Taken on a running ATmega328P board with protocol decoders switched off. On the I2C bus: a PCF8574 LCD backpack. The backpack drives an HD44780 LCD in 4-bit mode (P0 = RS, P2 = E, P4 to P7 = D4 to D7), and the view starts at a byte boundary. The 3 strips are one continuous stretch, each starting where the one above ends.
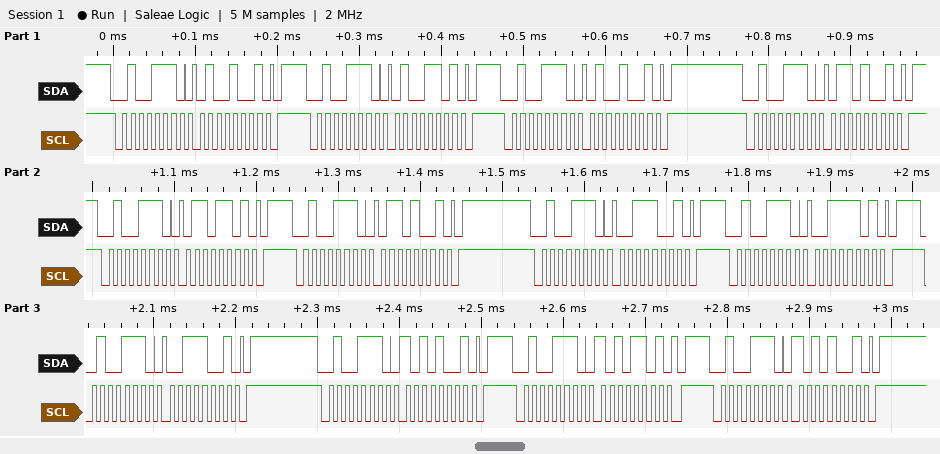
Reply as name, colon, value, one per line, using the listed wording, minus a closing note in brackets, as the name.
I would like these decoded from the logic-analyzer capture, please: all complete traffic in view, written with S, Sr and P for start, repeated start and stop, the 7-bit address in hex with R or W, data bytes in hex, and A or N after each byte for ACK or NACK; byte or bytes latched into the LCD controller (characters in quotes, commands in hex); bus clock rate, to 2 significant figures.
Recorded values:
all complete traffic in view, written with S, Sr and P for start, repeated start and stop, the 7-bit address in hex with R or W, data bytes in hex, and A or N after each byte for ACK or NACK: S 27W A 49 A P S 27W A 4D A P S 27W A 49 A P S 27W A 69 A P S 27W A 6D A P S 27W A 69 A P S 27W A 39 A P S 27W A 3D A P S 27W A 39 A P S 27W A A9 A P S 27W A AD A P S 27W A A9 A P
byte or bytes latched into the LCD controller: 'F' ':'
bus clock rate, to 2 significant figures: 100 kHz
